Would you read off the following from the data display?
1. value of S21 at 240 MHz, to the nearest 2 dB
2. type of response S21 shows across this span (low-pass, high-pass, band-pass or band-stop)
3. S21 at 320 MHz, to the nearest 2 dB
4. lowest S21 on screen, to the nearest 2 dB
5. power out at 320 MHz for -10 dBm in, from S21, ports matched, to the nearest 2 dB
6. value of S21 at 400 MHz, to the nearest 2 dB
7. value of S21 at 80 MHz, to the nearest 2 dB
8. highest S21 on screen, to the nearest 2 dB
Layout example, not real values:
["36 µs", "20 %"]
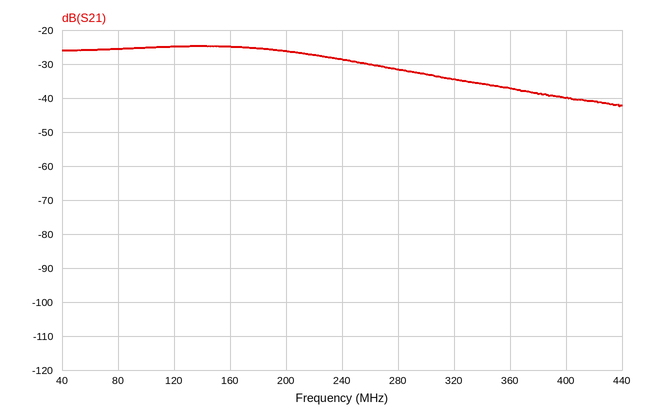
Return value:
["-28 dB", "low-pass", "-34 dB", "-42 dB", "-44 dBm", "-40 dB", "-26 dB", "-24 dB"]
